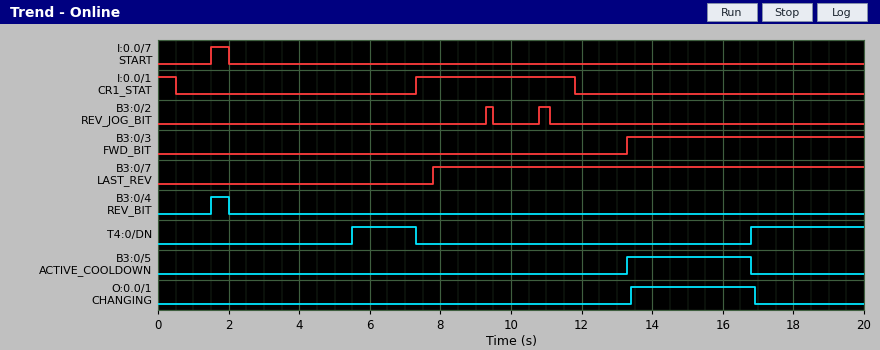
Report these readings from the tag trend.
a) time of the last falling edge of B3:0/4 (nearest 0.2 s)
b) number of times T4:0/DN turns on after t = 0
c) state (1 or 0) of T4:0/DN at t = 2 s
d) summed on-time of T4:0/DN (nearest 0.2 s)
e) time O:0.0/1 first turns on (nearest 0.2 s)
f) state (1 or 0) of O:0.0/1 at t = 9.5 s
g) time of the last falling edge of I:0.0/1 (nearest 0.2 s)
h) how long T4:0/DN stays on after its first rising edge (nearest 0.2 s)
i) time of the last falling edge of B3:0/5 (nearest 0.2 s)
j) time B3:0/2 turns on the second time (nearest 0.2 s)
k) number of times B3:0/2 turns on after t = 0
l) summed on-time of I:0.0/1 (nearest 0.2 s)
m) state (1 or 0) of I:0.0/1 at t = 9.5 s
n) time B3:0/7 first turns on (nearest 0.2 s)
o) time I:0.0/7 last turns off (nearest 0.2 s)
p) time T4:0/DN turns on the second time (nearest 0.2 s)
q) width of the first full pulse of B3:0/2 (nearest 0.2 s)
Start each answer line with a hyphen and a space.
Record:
- 2.0 s
- 2
- 0
- 5.0 s
- 13.4 s
- 0
- 11.8 s
- 1.8 s
- 16.8 s
- 10.8 s
- 2
- 5.0 s
- 1
- 7.8 s
- 2.0 s
- 16.8 s
- 0.2 s
